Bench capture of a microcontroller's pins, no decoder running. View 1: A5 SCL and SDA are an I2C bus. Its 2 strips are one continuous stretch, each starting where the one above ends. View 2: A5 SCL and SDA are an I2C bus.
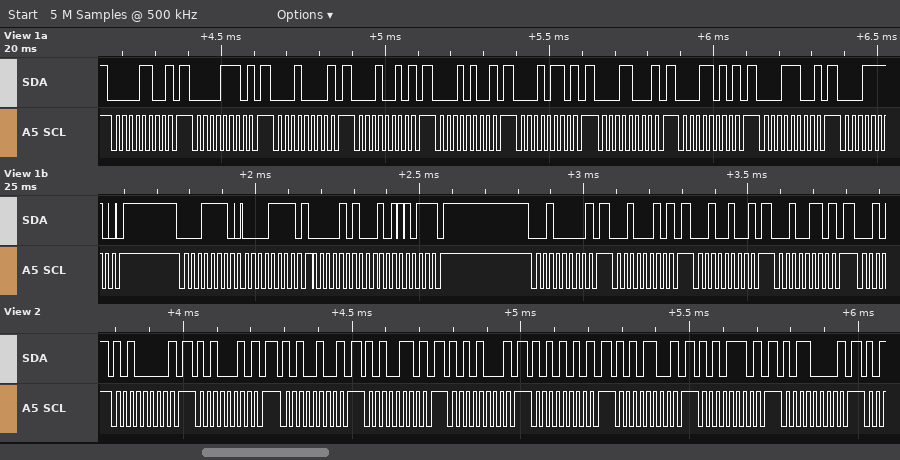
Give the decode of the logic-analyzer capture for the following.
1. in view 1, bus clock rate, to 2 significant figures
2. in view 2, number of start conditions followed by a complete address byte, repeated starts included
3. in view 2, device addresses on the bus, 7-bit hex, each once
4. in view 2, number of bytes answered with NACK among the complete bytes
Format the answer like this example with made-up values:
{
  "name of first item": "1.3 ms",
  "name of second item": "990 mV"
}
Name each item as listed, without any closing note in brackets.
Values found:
{
  "in view 1, bus clock rate, to 2 significant figures": "50 kHz",
  "in view 2, number of start conditions followed by a complete address byte, repeated starts included": "9",
  "in view 2, device addresses on the bus, 7-bit hex, each once": "0x50 0x51 0x52 0x53 0x54 0x55 0x56 0x57 0x58",
  "in view 2, number of bytes answered with NACK among the complete bytes": "9"
}
